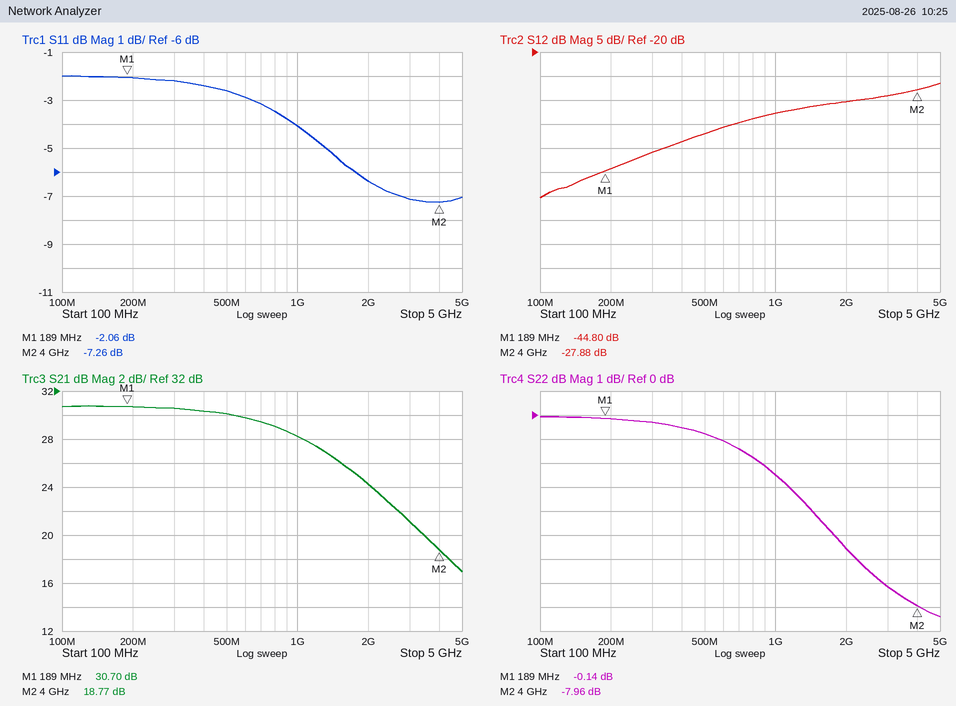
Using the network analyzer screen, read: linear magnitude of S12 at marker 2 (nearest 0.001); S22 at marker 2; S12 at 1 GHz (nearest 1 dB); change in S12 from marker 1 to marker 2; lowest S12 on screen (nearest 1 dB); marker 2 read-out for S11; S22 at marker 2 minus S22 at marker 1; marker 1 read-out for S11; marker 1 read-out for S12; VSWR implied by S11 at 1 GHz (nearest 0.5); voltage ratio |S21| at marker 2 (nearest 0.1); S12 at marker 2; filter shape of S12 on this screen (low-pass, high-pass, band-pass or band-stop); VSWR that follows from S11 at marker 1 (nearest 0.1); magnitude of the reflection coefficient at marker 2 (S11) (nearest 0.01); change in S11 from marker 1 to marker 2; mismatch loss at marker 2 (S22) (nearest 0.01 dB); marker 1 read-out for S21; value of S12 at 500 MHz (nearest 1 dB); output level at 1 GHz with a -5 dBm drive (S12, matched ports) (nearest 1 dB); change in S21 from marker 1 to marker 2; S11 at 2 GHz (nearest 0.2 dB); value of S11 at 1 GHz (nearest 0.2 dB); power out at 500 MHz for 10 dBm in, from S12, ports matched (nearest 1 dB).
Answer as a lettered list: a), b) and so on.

a) 0.040
b) -7.96 dB
c) -33 dB
d) 16.92 dB
e) -50 dB
f) -7.26 dB
g) -7.82 dB
h) -2.06 dB
i) -44.80 dB
j) 4.5
k) 8.7
l) -27.88 dB
m) high-pass
n) 8.5
o) 0.43
p) -5.20 dB
q) 0.76 dB
r) 30.70 dB
s) -37 dB
t) -38 dBm
u) -11.93 dB
v) -6.4 dB
w) -4.0 dB
x) -27 dBm
